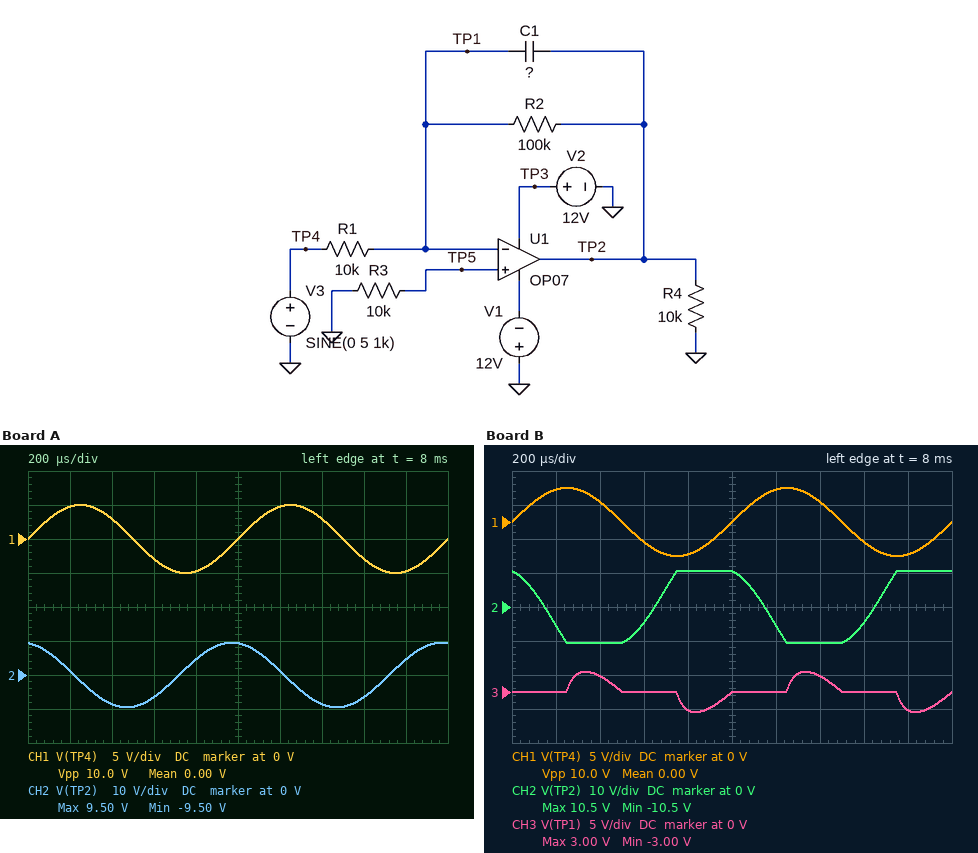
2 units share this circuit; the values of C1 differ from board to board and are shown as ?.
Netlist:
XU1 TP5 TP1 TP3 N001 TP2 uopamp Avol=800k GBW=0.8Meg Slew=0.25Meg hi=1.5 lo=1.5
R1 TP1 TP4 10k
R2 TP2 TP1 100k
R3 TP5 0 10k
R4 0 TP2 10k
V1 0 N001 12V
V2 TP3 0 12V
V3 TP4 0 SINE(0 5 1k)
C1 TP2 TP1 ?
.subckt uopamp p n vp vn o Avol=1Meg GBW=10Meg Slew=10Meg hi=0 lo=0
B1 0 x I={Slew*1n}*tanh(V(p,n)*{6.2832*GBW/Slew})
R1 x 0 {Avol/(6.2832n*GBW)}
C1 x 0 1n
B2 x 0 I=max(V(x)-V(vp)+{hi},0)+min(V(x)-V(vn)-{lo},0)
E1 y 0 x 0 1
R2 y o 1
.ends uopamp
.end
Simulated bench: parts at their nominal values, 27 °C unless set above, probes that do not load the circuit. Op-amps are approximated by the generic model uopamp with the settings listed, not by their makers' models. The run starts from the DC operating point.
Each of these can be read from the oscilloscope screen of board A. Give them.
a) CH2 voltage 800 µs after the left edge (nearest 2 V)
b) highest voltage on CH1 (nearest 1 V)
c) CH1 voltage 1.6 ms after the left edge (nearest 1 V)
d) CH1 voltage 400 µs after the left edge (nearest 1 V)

4 V
5 V
-3 V
3 V
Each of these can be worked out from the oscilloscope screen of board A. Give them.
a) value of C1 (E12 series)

8.2 nF
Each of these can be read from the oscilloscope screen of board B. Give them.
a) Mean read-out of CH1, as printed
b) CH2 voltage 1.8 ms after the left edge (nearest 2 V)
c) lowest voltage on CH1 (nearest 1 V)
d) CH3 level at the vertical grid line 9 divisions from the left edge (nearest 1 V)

0.00 V
10 V
-5 V
-3 V
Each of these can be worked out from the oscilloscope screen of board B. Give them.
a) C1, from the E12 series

3.9 nF
